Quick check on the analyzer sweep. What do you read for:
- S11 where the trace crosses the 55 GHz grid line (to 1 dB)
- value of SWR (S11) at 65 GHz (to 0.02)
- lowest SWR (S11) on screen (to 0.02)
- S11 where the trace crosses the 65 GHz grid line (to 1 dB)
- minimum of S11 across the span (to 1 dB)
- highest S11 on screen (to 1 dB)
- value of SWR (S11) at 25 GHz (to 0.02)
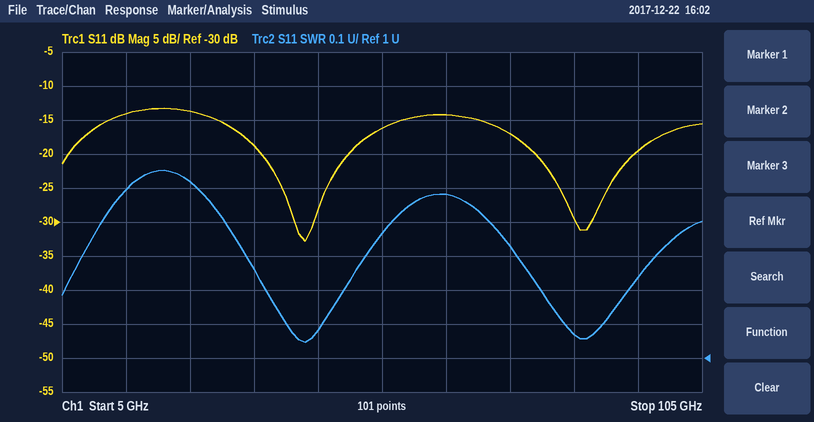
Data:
-16 dB
1.48
1.04
-14 dB
-33 dB
-13 dB
1.52
